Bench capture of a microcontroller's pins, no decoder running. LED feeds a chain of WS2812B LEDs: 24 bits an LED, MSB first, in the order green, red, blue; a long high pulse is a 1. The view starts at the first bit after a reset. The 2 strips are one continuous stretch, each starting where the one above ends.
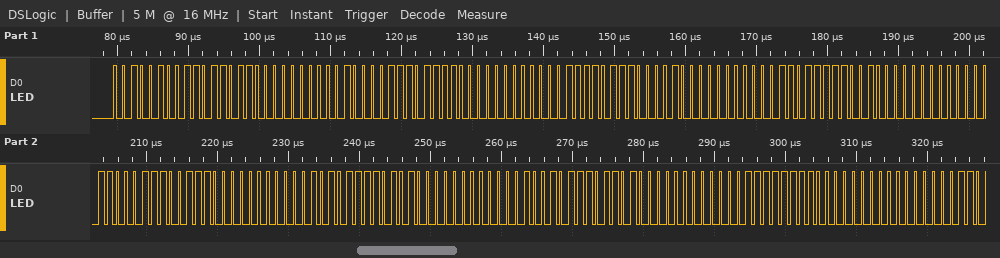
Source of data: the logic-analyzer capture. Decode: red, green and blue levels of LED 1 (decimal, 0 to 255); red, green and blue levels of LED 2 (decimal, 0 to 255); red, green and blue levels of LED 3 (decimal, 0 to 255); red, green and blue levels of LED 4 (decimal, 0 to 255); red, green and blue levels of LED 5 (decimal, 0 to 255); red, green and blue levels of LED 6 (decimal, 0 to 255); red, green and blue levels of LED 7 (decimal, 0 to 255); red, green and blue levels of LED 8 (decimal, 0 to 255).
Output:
219, 36, 0
222, 33, 0
225, 30, 0
228, 27, 0
231, 24, 0
234, 21, 0
237, 18, 0
240, 15, 0
